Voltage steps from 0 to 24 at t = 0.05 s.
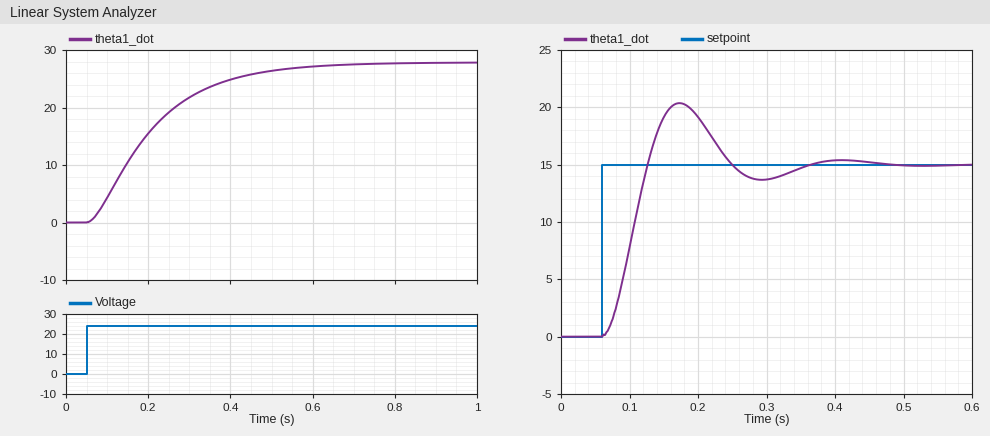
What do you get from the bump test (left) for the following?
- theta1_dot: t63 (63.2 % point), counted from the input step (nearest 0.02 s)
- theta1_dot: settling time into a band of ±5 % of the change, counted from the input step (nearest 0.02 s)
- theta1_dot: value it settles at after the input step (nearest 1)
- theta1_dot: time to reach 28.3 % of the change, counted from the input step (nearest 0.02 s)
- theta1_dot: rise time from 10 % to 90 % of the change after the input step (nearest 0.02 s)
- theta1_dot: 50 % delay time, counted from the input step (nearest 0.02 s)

0.18 s
0.46 s
28
0.08 s
0.32 s
0.14 s
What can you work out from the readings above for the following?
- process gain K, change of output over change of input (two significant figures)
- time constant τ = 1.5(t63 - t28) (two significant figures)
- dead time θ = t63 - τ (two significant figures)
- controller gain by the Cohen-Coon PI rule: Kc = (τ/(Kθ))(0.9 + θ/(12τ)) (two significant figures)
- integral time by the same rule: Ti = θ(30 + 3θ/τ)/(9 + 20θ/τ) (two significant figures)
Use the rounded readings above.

1.2
0.15 s
0.030 s
3.8
0.071 s
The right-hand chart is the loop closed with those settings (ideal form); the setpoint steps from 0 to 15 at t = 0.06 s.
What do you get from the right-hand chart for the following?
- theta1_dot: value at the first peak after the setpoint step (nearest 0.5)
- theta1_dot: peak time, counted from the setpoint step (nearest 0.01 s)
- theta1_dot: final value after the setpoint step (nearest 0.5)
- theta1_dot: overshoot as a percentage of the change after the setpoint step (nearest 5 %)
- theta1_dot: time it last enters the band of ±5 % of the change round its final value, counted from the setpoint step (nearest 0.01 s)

20.5
0.11 s
15.0
35 %
0.27 s
